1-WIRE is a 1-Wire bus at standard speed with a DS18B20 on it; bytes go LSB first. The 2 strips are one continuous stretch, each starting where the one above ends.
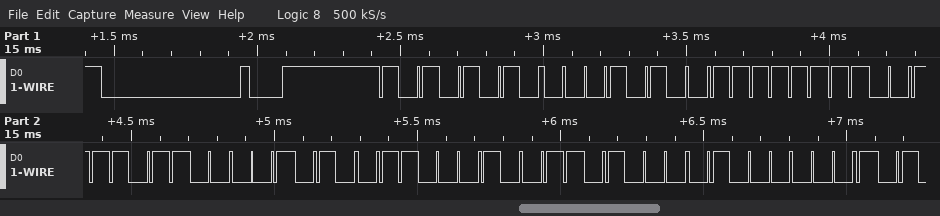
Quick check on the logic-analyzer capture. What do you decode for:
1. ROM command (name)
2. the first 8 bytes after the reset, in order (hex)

Match ROM
55 28 FF DC 50 46 16 02
